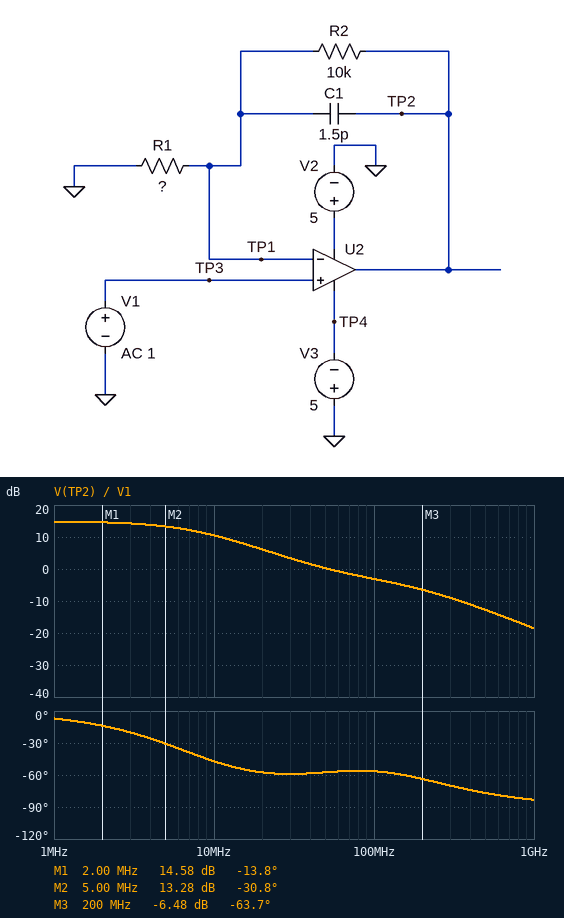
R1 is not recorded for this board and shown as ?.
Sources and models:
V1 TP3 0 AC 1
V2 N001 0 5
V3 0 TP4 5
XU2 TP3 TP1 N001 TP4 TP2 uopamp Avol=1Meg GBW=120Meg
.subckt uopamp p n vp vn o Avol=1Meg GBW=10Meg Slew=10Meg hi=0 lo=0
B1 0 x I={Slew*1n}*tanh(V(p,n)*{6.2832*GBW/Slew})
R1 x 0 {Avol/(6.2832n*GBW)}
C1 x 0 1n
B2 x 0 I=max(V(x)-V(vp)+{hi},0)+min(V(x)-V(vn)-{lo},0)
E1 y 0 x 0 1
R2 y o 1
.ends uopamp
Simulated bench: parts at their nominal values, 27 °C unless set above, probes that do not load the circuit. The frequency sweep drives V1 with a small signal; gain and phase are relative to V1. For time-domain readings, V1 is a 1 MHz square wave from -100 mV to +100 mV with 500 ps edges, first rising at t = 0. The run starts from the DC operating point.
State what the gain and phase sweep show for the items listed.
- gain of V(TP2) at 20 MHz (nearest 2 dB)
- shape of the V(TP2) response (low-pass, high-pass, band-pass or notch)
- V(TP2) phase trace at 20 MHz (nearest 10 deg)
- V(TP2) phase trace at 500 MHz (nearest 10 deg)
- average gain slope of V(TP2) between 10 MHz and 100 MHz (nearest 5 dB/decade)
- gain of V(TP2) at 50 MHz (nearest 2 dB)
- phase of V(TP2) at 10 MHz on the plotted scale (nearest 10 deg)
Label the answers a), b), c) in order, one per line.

a) 6 dB
b) low-pass
c) -60 deg
d) -80 deg
e) -15 dB/decade
f) 0 dB
g) -50 deg
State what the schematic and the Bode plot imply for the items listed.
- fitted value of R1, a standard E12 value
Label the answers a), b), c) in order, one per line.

a) 2.2 kΩ
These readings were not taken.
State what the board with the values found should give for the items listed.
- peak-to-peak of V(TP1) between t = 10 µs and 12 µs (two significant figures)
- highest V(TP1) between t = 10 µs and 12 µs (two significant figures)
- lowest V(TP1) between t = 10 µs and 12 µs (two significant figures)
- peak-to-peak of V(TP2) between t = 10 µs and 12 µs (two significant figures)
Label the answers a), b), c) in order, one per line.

a) 200 mV
b) 100 mV
c) -100 mV
d) 1.1 V
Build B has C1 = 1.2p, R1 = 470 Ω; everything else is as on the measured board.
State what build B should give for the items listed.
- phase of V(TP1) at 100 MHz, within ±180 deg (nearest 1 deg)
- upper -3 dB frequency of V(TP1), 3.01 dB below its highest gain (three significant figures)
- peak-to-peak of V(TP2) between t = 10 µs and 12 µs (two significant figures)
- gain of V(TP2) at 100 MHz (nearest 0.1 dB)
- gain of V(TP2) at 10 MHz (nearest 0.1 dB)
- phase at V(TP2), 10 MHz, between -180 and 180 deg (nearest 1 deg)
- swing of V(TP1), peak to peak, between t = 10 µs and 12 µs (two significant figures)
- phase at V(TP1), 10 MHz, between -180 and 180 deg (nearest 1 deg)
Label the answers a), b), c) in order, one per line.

a) -19 deg
b) 4.24 MHz
c) 4.4 V
d) -1.1 dB
e) 18.1 dB
f) -68 deg
g) 200 mV
h) -33 deg
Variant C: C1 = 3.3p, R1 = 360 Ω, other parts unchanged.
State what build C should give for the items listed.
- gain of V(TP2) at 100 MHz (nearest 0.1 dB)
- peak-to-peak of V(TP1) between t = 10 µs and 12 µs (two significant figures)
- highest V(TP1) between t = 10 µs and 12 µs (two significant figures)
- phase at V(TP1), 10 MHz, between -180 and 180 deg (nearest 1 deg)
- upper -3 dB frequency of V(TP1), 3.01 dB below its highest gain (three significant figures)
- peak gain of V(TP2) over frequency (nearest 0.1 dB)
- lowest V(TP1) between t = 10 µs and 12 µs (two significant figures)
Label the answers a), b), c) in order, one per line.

a) -2.6 dB
b) 180 mV
c) 91 mV
d) -15 deg
e) 3.01 MHz
f) 29.2 dB
g) -91 mV
